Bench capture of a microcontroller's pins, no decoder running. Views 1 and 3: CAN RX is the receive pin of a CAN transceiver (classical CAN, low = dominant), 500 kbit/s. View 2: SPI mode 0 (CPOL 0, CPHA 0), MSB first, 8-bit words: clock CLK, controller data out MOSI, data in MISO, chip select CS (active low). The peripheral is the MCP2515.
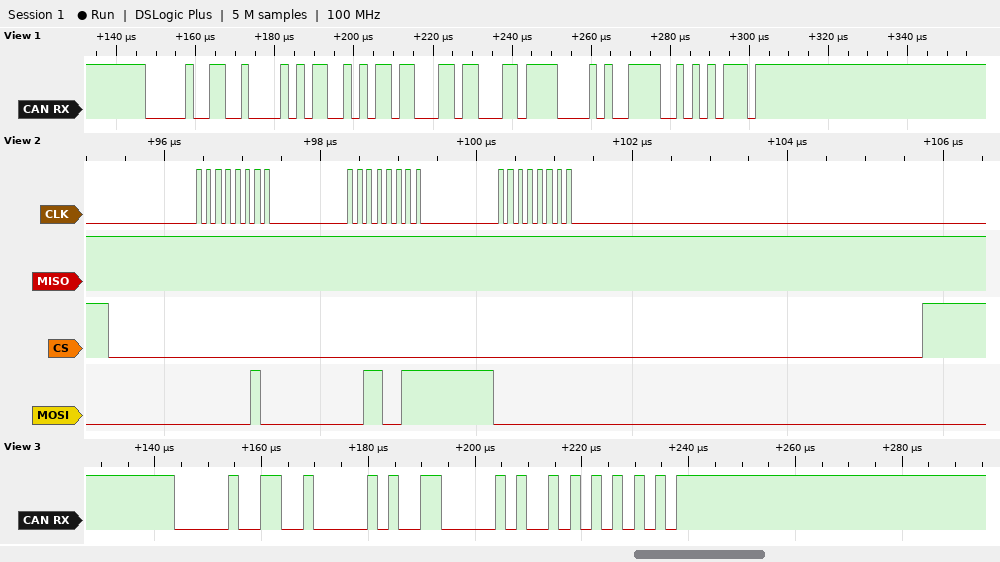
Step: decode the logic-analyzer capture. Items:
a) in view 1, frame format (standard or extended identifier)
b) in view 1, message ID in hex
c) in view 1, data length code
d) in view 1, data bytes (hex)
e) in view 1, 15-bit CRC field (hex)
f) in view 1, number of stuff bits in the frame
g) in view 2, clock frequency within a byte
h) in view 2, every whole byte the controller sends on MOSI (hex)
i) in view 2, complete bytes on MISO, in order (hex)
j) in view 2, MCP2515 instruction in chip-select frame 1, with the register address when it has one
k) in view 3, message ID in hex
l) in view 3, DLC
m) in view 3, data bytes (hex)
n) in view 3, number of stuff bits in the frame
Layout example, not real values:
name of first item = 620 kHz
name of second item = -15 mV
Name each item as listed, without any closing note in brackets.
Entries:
in view 1, frame format = standard
in view 1, message ID in hex = 0x019
in view 1, data length code = 5
in view 1, data bytes = 65 6C 6C 6F 0A
in view 1, 15-bit CRC field = 0x3CAB
in view 1, number of stuff bits in the frame = 1
in view 2, clock frequency within a byte = 8 MHz
in view 2, every whole byte the controller sends on MOSI = 02 33 00
in view 2, complete bytes on MISO, in order = FF FF FF
in view 2, MCP2515 instruction in chip-select frame 1, with the register address when it has one = WRITE 0x33
in view 3, message ID in hex = 0x019
in view 3, DLC = 1
in view 3, data bytes = 30
in view 3, number of stuff bits in the frame = 3
